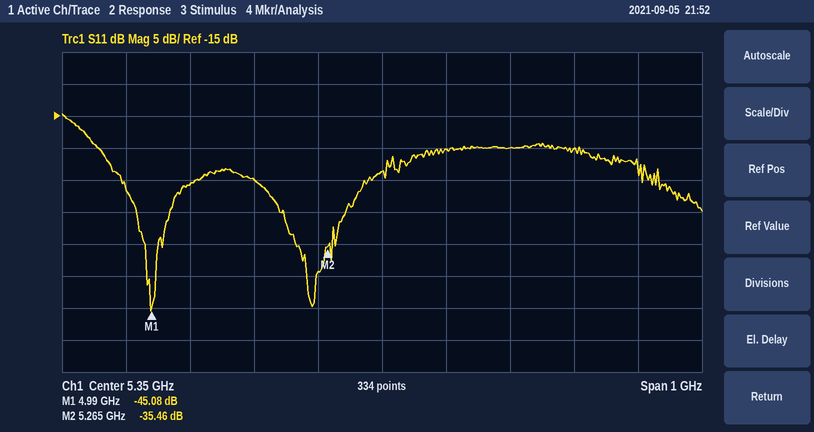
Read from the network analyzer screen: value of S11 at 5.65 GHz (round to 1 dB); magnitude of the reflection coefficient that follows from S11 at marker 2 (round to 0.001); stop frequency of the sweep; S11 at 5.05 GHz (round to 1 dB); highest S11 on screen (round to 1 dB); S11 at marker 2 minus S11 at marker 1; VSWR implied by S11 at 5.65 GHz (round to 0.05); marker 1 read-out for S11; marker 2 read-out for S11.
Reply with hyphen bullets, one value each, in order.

- -20 dB
- 0.017
- 5.85 GHz
- -26 dB
- -15 dB
- 9.62 dB
- 1.20
- -45.08 dB
- -35.46 dB
